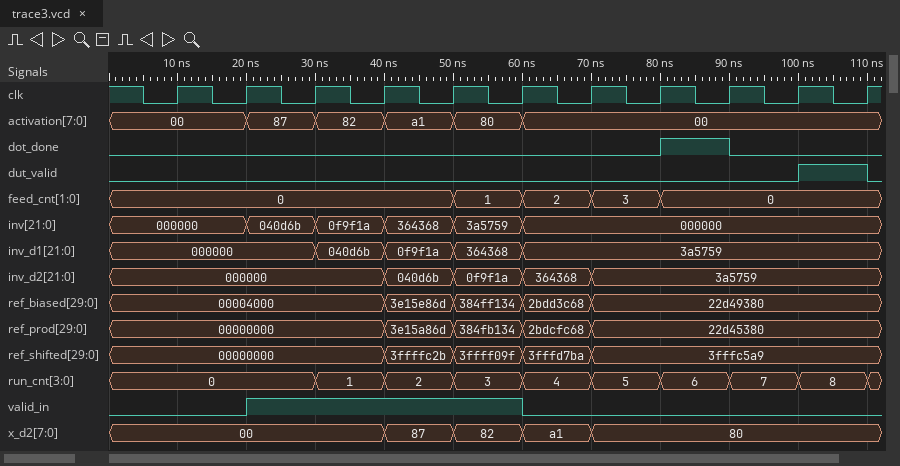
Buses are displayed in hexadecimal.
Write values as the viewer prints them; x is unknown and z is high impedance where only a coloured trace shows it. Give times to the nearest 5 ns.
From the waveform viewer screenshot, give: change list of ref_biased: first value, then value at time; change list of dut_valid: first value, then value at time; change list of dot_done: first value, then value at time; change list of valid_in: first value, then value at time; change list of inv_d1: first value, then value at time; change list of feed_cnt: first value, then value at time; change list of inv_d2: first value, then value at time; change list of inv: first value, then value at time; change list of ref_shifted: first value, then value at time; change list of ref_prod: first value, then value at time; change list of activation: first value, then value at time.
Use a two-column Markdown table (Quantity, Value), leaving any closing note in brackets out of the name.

| Quantity | Value |
|---|---|
| change list of ref_biased: first value, then value at time | 00004000, 3e15e86d at 40 ns, 384ff134 at 50 ns, 2bdd3c68 at 60 ns, 22d49380 at 70 ns |
| change list of dut_valid: first value, then value at time | 0, 1 at 100 ns, 0 at 110 ns |
| change list of dot_done: first value, then value at time | 0, 1 at 80 ns, 0 at 90 ns |
| change list of valid_in: first value, then value at time | 0, 1 at 20 ns, 0 at 60 ns |
| change list of inv_d1: first value, then value at time | 000000, 040d6b at 30 ns, 0f9f1a at 40 ns, 364368 at 50 ns, 3a5759 at 60 ns |
| change list of feed_cnt: first value, then value at time | 0, 1 at 50 ns, 2 at 60 ns, 3 at 70 ns, 0 at 80 ns |
| change list of inv_d2: first value, then value at time | 000000, 040d6b at 40 ns, 0f9f1a at 50 ns, 364368 at 60 ns, 3a5759 at 70 ns |
| change list of inv: first value, then value at time | 000000, 040d6b at 20 ns, 0f9f1a at 30 ns, 364368 at 40 ns, 3a5759 at 50 ns, 000000 at 60 ns |
| change list of ref_shifted: first value, then value at time | 00000000, 3ffffc2b at 40 ns, 3ffff09f at 50 ns, 3fffd7ba at 60 ns, 3fffc5a9 at 70 ns |
| change list of ref_prod: first value, then value at time | 00000000, 3e15a86d at 40 ns, 384fb134 at 50 ns, 2bdcfc68 at 60 ns, 22d45380 at 70 ns |
| change list of activation: first value, then value at time | 00, 87 at 20 ns, 82 at 30 ns, a1 at 40 ns, 80 at 50 ns, 00 at 60 ns |
